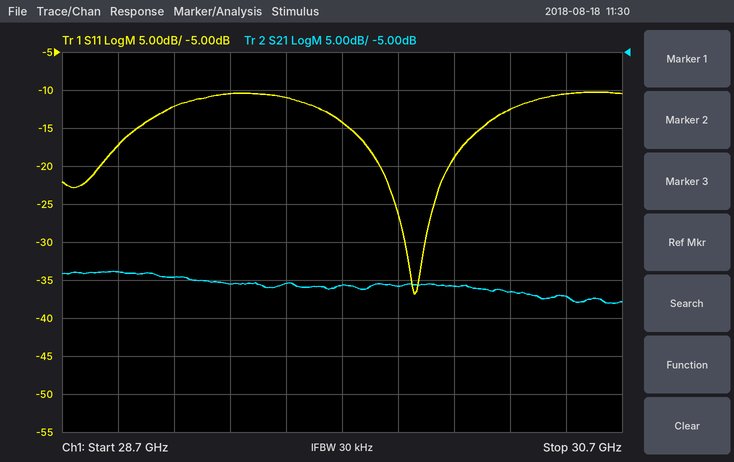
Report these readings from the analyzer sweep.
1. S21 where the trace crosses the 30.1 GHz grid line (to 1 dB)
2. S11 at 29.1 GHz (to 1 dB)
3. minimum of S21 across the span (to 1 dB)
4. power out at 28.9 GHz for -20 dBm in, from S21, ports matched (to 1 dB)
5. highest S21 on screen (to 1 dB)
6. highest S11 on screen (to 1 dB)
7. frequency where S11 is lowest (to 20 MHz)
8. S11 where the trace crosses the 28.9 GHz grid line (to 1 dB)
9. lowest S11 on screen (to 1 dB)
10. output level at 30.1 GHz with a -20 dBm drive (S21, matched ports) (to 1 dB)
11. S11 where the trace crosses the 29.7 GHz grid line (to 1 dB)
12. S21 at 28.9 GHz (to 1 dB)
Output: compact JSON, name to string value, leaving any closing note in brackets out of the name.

{"S21 where the trace crosses the 30.1 GHz grid line": "-36 dB", "S11 at 29.1 GHz": "-12 dB", "minimum of S21 across the span": "-38 dB", "power out at 28.9 GHz for -20 dBm in, from S21, ports matched": "-54 dBm", "highest S21 on screen": "-34 dB", "highest S11 on screen": "-10 dB", "frequency where S11 is lowest": "29.96 GHz", "S11 where the trace crosses the 28.9 GHz grid line": "-17 dB", "lowest S11 on screen": "-37 dB", "output level at 30.1 GHz with a -20 dBm drive (S21, matched ports)": "-56 dBm", "S11 where the trace crosses the 29.7 GHz grid line": "-14 dB", "S21 at 28.9 GHz": "-34 dB"}
